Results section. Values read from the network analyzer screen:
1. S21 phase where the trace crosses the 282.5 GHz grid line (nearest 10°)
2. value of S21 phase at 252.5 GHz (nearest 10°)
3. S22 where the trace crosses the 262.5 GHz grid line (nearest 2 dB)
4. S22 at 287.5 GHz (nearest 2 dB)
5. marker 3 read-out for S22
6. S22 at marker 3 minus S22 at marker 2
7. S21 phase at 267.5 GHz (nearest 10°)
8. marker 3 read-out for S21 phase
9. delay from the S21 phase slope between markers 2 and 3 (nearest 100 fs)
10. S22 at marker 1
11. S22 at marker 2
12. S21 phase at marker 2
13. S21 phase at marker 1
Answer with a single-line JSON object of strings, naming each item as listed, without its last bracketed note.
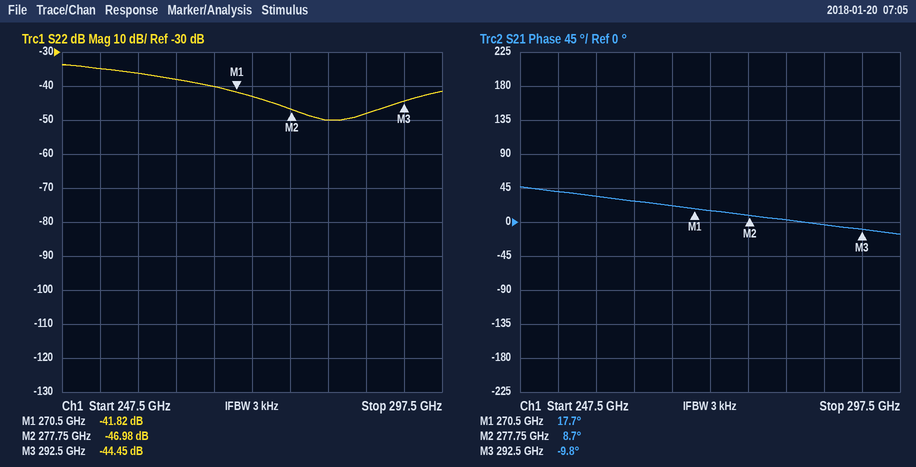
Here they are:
{"S21 phase where the trace crosses the 282.5 GHz grid line": "0°", "value of S21 phase at 252.5 GHz": "40°", "S22 where the trace crosses the 262.5 GHz grid line": "-38 dB", "S22 at 287.5 GHz": "-48 dB", "marker 3 read-out for S22": "-44.45 dB", "S22 at marker 3 minus S22 at marker 2": "2.53 dB", "S21 phase at 267.5 GHz": "20°", "marker 3 read-out for S21 phase": "-9.8°", "delay from the S21 phase slope between markers 2 and 3": "3.5 ps", "S22 at marker 1": "-41.82 dB", "S22 at marker 2": "-46.98 dB", "S21 phase at marker 2": "8.7°", "S21 phase at marker 1": "17.7°"}
